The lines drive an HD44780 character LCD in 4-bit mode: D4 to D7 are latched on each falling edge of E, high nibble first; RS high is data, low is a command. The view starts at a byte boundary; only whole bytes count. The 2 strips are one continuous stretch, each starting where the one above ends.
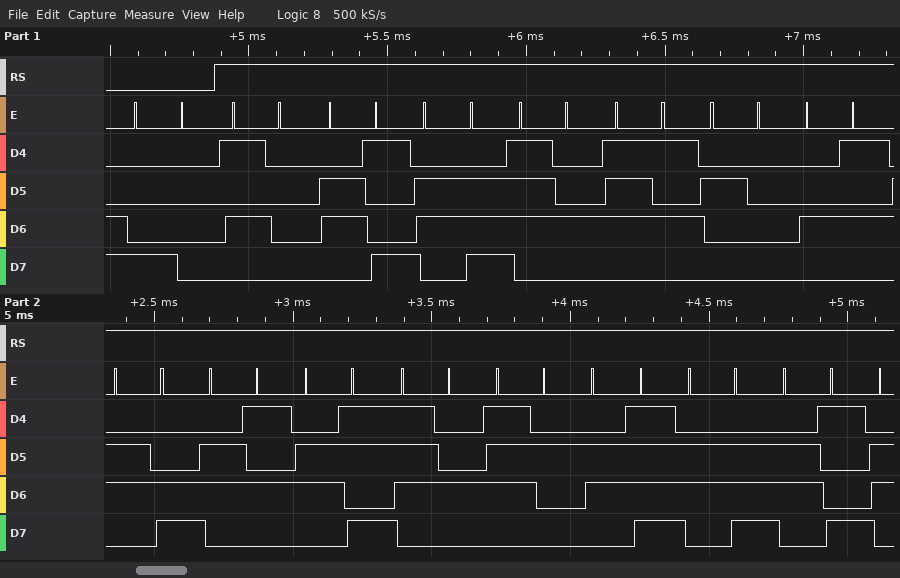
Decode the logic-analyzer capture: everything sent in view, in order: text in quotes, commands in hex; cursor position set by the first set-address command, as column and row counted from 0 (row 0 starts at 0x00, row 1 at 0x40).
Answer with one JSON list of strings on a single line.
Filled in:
["0x80 \"Pintu Elektroni\"", "column 0, row 0"]
